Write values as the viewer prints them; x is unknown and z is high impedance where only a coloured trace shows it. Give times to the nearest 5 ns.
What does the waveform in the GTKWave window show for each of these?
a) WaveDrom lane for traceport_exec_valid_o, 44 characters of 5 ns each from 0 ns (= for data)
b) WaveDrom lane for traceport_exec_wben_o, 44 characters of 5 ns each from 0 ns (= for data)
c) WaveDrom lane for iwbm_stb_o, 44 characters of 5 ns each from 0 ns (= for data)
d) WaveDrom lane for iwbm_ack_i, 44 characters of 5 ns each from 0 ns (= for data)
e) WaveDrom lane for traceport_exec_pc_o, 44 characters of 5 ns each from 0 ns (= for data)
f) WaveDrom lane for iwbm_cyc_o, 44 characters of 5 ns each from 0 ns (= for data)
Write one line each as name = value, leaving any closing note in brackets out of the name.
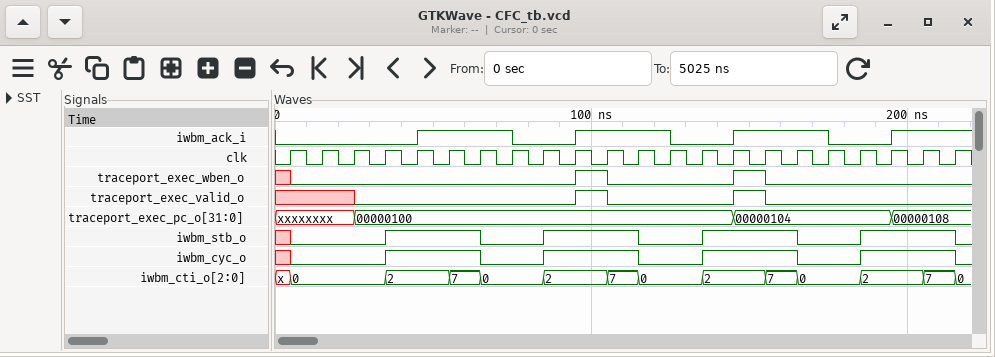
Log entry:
WaveDrom lane for traceport_exec_valid_o, 44 characters of 5 ns each from 0 ns = {name: 'traceport_exec_valid_o', wave: 'x....0.............1.0.......1.0............'}
WaveDrom lane for traceport_exec_wben_o, 44 characters of 5 ns each from 0 ns = {name: 'traceport_exec_wben_o', wave: 'x0.................1.0.......1.0............'}
WaveDrom lane for iwbm_stb_o, 44 characters of 5 ns each from 0 ns = {name: 'iwbm_stb_o', wave: 'x0.....1.....0...1.....0...1.....0...1.....0'}
WaveDrom lane for iwbm_ack_i, 44 characters of 5 ns each from 0 ns = {name: 'iwbm_ack_i', wave: '0........1.....0...1.....0...1.....0...1....'}
WaveDrom lane for traceport_exec_pc_o, 44 characters of 5 ns each from 0 ns = {name: 'traceport_exec_pc_o', wave: 'x....=.......................=.........=....', data: '00000100 00000104 00000108'}
WaveDrom lane for iwbm_cyc_o, 44 characters of 5 ns each from 0 ns = {name: 'iwbm_cyc_o', wave: 'x0.....1.....0...1.....0...1.....0...1.....0'}
